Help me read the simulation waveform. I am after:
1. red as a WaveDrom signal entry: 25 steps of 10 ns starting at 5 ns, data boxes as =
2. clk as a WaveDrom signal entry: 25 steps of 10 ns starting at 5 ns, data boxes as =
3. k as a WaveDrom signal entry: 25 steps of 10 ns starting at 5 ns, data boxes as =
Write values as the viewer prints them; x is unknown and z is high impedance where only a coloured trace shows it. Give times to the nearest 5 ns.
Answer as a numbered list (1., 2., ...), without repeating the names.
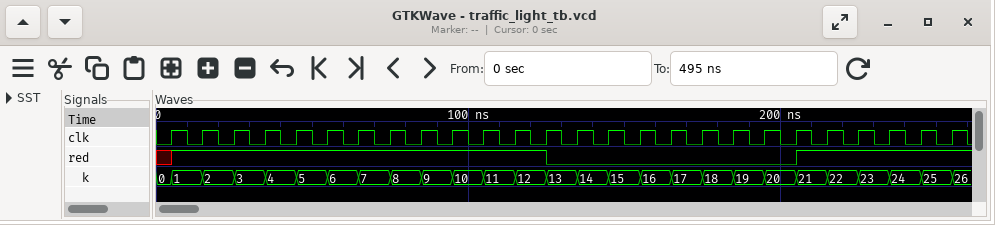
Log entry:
1. {name: 'red', wave: '1...........0.......1....'}
2. {name: 'clk', wave: 'p........................'}
3. {name: 'k', wave: '=========================', data: '1 2 3 4 5 6 7 8 9 10 11 12 13 14 15 16 17 18 19 20 21 22 23 24 25'}
